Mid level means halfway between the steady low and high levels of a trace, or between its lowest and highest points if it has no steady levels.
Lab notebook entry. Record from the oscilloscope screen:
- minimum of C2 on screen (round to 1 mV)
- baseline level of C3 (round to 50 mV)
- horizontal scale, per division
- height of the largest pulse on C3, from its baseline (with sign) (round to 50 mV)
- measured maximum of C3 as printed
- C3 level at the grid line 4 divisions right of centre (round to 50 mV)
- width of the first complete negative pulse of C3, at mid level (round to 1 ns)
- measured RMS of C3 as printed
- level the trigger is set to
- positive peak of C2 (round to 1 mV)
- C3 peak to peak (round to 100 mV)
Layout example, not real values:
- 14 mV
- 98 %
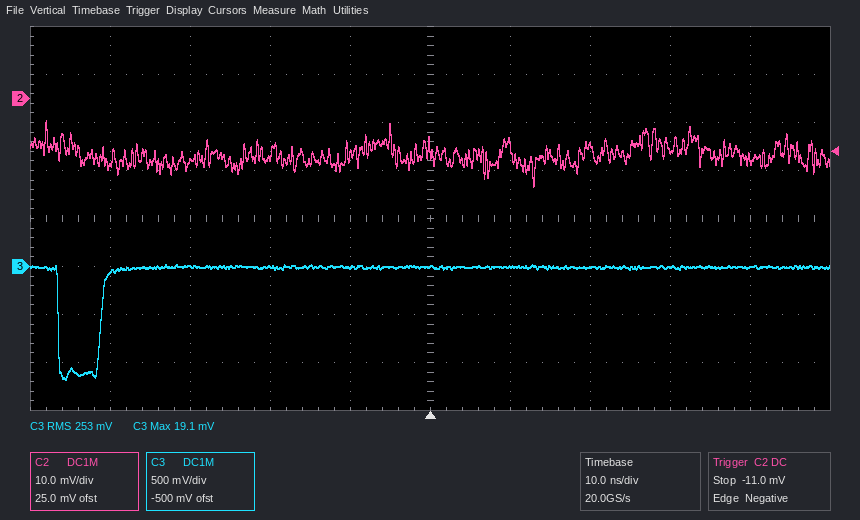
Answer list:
- -18 mV
- 0 mV
- 10 ns
- -1.15 V
- 19.1 mV
- 0 mV
- 5 ns
- 253 mV
- -11.0 mV
- -5 mV
- 1.20 V
